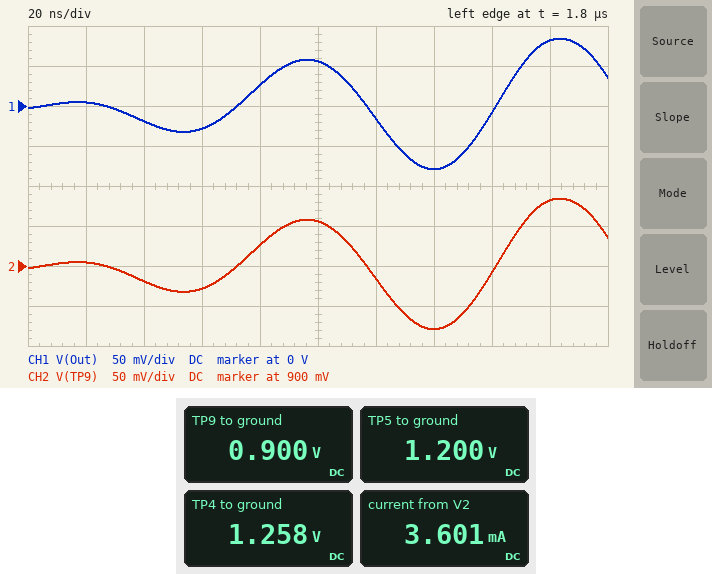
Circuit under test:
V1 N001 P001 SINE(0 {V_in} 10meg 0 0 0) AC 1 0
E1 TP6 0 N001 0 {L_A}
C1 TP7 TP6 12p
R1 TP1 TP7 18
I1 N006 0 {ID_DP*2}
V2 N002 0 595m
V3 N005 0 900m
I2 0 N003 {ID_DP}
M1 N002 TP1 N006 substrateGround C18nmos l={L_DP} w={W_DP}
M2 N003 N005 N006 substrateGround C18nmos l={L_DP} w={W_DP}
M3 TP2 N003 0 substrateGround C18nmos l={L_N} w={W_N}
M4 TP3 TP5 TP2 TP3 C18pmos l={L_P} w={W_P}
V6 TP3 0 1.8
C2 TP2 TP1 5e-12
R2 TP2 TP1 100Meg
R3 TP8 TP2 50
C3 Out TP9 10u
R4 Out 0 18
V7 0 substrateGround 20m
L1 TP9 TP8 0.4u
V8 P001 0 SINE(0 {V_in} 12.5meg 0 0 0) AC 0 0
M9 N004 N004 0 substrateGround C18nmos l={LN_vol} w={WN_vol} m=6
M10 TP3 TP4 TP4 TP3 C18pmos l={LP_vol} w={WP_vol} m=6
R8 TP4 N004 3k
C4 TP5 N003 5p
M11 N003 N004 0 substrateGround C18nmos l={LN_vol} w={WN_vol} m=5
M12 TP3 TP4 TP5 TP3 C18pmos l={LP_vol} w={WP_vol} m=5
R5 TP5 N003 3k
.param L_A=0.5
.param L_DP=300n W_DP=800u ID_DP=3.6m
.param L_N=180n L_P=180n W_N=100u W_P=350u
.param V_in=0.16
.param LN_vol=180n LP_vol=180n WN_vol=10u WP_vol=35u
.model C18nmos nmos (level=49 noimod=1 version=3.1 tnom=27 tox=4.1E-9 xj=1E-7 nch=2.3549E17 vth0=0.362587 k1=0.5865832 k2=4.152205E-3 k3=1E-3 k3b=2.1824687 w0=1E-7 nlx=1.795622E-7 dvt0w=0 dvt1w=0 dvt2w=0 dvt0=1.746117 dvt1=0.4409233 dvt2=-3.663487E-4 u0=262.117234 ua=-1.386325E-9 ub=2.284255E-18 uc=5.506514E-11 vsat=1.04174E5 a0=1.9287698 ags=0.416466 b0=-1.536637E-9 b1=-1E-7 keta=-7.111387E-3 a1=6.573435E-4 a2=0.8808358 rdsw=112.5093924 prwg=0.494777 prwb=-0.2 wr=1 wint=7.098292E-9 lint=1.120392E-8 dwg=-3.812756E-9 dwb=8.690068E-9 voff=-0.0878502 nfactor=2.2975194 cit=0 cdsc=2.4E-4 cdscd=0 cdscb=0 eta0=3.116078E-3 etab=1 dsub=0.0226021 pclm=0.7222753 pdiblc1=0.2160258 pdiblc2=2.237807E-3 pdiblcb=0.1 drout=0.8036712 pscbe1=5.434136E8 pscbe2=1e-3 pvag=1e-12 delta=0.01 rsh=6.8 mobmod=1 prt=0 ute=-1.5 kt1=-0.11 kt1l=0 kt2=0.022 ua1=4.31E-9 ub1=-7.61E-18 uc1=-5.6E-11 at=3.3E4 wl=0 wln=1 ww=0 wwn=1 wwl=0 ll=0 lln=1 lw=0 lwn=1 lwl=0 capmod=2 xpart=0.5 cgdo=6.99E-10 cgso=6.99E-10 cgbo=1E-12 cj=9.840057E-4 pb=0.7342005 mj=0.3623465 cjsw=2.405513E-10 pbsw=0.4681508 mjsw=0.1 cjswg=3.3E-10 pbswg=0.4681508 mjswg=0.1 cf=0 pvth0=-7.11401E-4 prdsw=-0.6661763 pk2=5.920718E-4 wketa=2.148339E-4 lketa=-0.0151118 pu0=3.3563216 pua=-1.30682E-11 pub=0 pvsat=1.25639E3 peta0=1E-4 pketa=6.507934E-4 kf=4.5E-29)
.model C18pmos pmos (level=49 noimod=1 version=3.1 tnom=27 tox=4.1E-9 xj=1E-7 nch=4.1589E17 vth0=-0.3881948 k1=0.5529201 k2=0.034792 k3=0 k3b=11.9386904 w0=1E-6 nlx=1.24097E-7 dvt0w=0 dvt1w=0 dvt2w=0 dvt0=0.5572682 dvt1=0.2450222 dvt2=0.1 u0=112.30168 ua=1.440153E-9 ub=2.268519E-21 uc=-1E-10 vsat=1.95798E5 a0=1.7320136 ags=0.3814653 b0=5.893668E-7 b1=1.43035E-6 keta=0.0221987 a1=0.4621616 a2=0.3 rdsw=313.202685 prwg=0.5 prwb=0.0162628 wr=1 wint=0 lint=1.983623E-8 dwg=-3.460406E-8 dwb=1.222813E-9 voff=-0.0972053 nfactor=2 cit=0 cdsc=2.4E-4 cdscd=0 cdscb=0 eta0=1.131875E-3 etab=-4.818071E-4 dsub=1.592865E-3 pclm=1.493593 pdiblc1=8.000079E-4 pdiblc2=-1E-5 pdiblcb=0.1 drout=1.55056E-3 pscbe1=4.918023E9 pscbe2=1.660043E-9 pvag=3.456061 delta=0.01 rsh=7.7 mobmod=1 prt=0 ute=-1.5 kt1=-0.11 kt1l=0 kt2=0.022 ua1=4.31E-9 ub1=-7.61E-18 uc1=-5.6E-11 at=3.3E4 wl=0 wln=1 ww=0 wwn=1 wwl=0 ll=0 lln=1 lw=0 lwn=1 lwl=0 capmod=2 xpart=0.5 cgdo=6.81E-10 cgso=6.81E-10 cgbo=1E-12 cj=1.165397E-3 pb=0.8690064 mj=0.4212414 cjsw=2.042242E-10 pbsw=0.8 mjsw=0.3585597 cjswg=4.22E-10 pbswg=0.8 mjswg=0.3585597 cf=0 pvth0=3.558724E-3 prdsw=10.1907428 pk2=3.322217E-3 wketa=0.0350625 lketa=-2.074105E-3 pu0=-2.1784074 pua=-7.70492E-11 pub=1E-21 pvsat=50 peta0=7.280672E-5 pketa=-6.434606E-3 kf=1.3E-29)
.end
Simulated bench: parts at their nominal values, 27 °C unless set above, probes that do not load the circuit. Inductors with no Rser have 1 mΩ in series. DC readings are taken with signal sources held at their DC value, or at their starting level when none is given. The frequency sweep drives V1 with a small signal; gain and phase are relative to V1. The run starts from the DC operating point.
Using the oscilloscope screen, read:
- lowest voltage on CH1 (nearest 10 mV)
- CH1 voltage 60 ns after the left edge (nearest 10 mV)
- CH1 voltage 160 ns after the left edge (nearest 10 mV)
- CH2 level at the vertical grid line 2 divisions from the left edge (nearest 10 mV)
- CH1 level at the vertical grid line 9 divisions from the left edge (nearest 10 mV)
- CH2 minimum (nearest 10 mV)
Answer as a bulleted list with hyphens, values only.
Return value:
- -80 mV
- -30 mV
- -10 mV
- 880 mV
- 80 mV
- 820 mV
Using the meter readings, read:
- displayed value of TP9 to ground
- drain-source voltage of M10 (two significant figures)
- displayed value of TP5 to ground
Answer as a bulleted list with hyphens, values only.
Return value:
- 0.900 V
- 540 mV
- 1.200 V
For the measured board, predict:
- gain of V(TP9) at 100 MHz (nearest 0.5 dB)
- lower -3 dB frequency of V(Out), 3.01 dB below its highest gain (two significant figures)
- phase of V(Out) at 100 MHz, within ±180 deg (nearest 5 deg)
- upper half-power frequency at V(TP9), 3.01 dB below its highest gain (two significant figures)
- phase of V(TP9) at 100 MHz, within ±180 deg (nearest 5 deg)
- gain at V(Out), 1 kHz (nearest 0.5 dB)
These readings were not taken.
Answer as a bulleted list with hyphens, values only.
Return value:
- -22.0 dB
- 420 Hz
- 95 deg
- 1.1 kHz
- 95 deg
- -11.0 dB
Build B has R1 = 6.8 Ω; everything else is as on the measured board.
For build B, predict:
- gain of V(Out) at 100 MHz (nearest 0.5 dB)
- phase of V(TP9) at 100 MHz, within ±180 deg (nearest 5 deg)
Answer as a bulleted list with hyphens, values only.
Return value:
- -21.5 dB
- 100 deg
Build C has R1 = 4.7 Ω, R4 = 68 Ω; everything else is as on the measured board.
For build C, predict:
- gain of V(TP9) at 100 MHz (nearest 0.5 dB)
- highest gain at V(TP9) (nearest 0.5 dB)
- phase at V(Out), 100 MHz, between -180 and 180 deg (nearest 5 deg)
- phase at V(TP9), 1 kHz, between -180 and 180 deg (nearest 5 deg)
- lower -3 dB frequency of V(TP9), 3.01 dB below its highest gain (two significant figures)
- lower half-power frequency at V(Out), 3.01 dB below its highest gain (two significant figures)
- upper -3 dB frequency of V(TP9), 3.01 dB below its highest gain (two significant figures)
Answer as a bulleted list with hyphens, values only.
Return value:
- -10.5 dB
- -3.5 dB
- 110 deg
- -170 deg
- 210 Hz
- 360 Hz
- 47 MHz
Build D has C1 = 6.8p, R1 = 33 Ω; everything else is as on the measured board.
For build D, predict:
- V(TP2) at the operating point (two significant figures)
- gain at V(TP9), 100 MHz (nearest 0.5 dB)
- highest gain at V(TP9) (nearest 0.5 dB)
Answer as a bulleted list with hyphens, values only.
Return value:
- 900 mV
- -26.5 dB
- -10.5 dB
